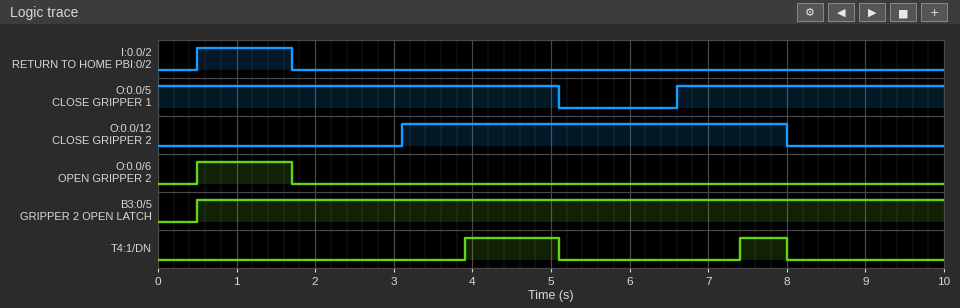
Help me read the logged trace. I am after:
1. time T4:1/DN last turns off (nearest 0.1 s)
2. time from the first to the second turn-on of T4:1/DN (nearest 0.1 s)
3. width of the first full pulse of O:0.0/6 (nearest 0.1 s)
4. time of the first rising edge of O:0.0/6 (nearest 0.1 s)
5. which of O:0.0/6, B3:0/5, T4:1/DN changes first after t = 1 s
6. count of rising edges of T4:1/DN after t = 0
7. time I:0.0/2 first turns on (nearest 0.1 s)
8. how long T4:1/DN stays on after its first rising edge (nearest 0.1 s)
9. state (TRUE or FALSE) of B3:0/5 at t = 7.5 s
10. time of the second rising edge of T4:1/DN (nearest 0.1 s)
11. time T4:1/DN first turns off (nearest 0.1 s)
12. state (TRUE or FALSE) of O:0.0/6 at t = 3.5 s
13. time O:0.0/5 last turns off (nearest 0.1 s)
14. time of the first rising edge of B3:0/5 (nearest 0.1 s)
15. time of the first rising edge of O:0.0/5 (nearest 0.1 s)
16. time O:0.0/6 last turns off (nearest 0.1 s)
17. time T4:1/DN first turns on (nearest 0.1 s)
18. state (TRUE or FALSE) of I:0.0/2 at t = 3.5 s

8.0 s
3.5 s
1.2 s
0.5 s
O:0.0/6
2
0.5 s
1.2 s
TRUE
7.4 s
5.1 s
FALSE
5.1 s
0.5 s
6.6 s
1.7 s
3.9 s
FALSE
